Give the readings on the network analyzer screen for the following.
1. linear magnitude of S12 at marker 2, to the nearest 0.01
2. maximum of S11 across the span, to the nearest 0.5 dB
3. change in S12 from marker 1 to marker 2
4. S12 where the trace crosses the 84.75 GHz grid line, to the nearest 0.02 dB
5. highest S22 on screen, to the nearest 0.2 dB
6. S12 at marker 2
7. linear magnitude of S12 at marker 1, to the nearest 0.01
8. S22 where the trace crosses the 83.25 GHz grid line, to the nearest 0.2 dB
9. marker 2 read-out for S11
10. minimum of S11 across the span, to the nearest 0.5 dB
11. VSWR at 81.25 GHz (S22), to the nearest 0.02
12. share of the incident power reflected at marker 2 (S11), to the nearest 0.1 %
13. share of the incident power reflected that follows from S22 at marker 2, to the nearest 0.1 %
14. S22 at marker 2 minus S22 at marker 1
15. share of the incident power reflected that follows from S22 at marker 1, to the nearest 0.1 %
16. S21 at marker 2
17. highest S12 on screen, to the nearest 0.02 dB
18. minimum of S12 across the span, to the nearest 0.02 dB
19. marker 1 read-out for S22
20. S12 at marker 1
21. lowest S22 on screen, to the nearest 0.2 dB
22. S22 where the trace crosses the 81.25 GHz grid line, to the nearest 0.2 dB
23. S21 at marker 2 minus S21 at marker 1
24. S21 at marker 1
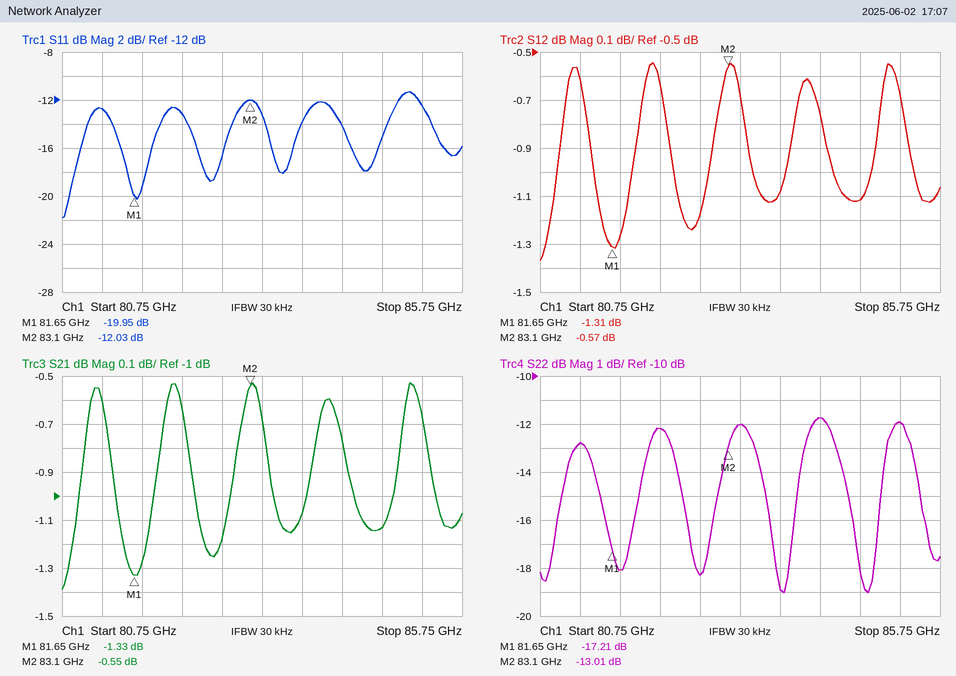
0.94
-11.5 dB
0.74 dB
-1.12 dB
-11.8 dB
-0.57 dB
0.86
-12.0 dB
-12.03 dB
-22.0 dB
1.60
6.3 %
5.0 %
4.20 dB
1.9 %
-0.55 dB
-0.54 dB
-1.36 dB
-17.21 dB
-1.31 dB
-19.0 dB
-12.8 dB
0.78 dB
-1.33 dB
